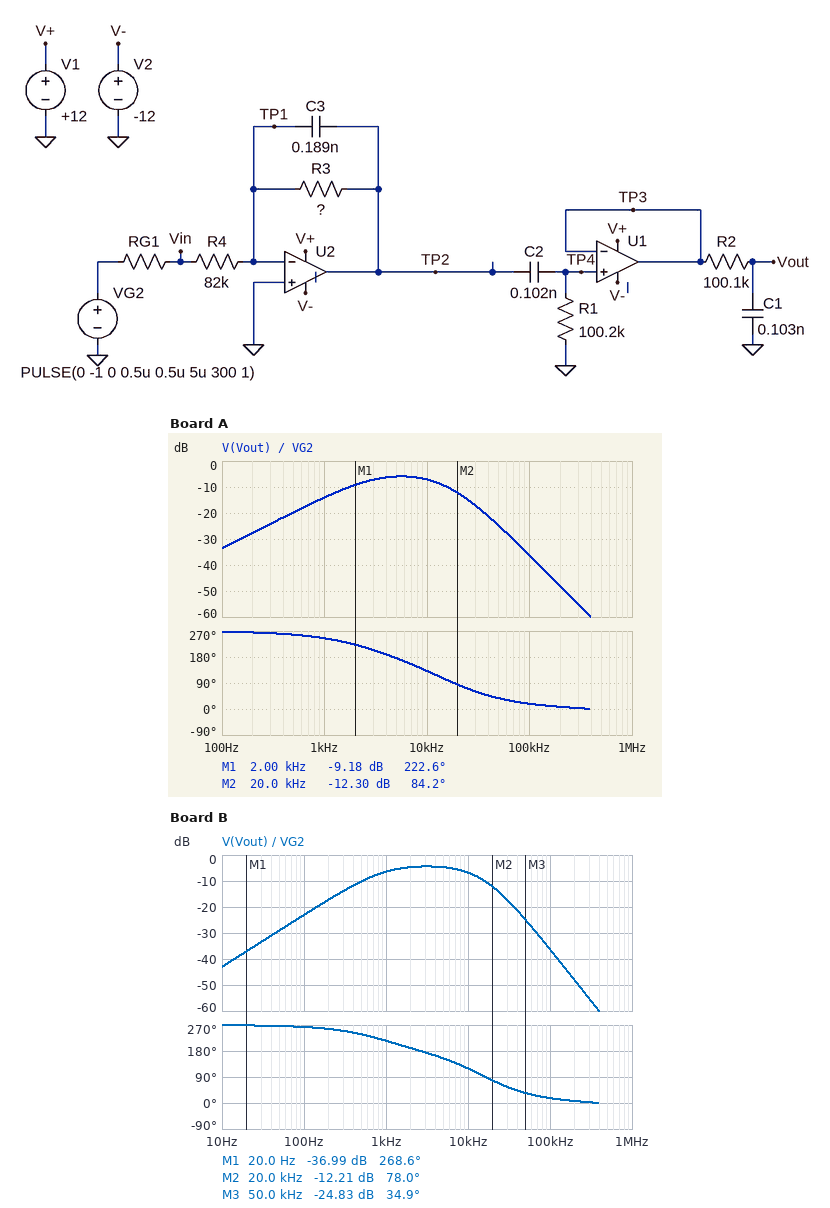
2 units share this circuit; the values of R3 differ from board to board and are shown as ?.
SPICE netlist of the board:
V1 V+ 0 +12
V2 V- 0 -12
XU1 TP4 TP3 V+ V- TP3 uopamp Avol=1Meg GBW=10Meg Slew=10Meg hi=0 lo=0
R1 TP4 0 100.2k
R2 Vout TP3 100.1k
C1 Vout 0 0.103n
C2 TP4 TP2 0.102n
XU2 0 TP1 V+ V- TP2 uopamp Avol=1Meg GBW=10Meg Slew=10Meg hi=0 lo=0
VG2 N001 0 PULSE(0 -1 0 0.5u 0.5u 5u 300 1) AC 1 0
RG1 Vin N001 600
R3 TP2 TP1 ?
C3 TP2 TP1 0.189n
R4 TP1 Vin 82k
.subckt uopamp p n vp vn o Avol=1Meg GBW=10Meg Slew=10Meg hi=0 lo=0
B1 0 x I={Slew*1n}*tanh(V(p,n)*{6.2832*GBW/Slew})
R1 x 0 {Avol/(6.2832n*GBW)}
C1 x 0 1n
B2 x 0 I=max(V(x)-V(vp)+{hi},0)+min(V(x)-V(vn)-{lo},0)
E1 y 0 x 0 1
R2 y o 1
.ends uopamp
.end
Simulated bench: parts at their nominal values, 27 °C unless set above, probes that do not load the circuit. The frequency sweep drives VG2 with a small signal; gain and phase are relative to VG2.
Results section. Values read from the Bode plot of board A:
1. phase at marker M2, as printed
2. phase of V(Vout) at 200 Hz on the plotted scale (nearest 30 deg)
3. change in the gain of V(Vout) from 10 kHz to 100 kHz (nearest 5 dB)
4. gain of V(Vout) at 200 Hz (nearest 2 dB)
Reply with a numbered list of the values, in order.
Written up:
1. 84.2 deg
2. 270 deg
3. -30 dB
4. -28 dB
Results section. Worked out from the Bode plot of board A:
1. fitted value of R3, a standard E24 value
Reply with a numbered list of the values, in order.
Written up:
1. 270 kΩ
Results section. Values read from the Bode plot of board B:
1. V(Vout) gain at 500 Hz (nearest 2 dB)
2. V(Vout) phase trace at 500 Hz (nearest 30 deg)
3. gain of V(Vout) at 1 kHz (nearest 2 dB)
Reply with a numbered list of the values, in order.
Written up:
1. -10 dB
2. 240 deg
3. -6 dB
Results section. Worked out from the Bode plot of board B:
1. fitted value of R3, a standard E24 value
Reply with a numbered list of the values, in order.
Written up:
1. 910 kΩ
